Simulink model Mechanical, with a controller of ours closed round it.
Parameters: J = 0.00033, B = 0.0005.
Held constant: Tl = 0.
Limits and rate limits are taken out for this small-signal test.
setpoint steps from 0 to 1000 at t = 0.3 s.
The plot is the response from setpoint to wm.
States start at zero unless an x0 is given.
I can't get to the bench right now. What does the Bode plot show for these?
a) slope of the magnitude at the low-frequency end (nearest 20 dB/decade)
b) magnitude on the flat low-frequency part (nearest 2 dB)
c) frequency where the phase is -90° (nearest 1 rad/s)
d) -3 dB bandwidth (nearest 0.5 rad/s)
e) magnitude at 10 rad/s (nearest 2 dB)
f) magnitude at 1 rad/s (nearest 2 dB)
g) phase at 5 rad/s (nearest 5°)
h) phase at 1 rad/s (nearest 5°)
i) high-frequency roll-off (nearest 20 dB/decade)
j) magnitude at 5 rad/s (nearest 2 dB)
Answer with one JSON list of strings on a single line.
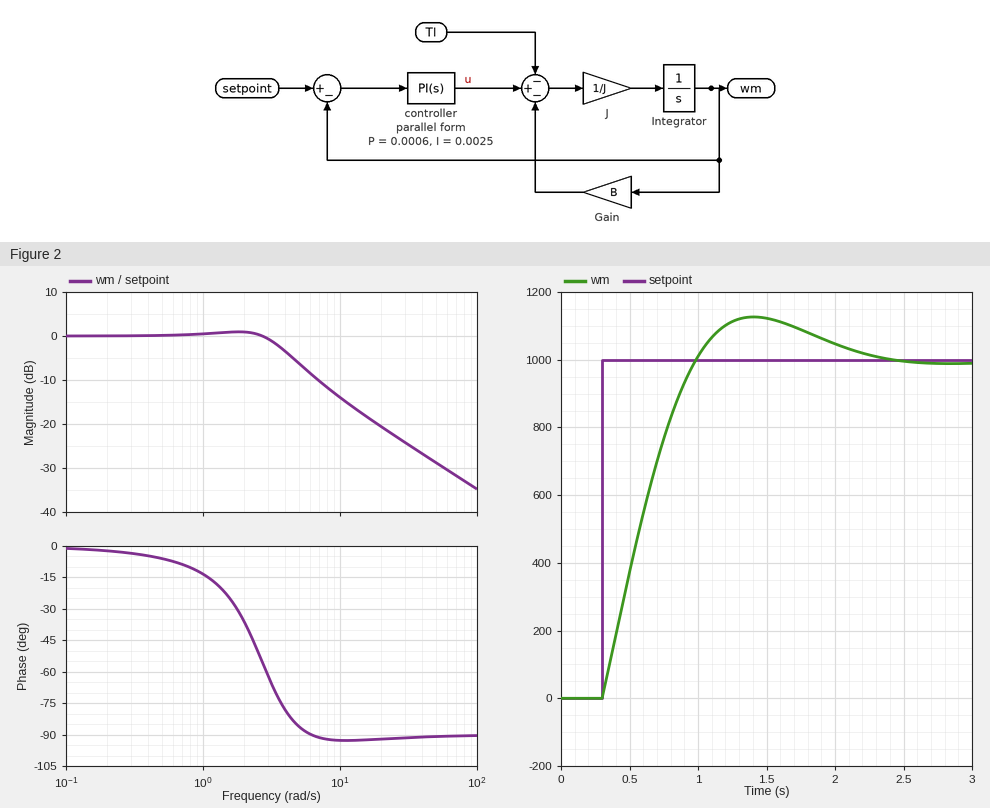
["0 dB/decade", "0 dB", "6 rad/s", "4.0 rad/s", "-14 dB", "0 dB", "-85°", "-15°", "-20 dB/decade", "-6 dB"]
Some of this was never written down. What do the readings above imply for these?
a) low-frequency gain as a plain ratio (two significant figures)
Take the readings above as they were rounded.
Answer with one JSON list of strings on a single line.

["1.0"]
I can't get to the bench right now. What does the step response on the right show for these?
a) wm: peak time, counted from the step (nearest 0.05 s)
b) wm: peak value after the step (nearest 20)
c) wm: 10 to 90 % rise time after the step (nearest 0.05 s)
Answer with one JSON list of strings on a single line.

["1.10 s", "1120", "0.50 s"]
